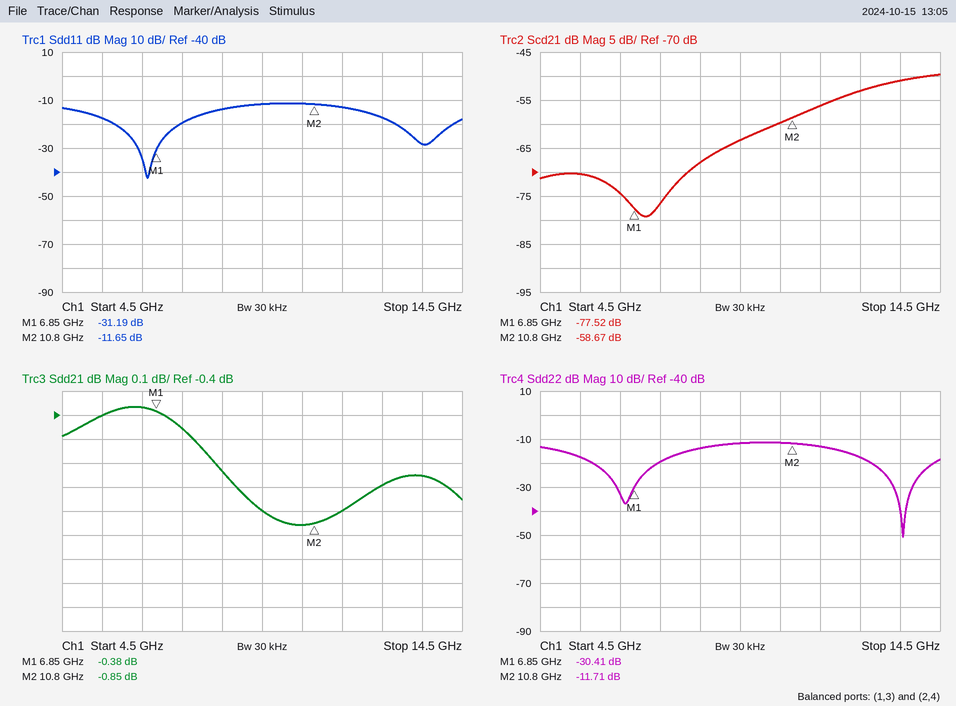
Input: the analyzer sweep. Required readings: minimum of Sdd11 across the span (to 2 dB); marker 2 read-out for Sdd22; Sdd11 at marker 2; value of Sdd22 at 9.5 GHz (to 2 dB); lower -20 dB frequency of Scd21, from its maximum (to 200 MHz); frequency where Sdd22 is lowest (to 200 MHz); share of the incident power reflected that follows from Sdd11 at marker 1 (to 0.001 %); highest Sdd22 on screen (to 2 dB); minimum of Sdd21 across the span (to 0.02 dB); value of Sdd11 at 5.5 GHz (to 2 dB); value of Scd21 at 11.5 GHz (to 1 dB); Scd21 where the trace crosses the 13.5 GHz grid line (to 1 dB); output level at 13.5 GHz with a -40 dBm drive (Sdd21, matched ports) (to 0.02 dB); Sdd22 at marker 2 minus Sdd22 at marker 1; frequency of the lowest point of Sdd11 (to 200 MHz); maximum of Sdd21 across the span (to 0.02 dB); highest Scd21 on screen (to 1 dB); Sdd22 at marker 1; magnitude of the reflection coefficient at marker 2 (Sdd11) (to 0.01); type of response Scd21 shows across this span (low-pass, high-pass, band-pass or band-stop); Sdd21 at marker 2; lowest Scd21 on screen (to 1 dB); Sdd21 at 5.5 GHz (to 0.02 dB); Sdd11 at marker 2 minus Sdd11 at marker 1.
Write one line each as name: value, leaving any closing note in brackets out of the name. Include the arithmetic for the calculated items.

minimum of Sdd11 across the span: -42 dB
marker 2 read-out for Sdd22: -11.71 dB
Sdd11 at marker 2: -11.65 dB
value of Sdd22 at 9.5 GHz: -12 dB
lower -20 dB frequency of Scd21, from its maximum: 8.2 GHz
frequency where Sdd22 is lowest: 13.6 GHz
share of the incident power reflected that follows from Sdd11 at marker 1: 10^(-31.19/10) ≈ 0.076 %
highest Sdd22 on screen: -12 dB
minimum of Sdd21 across the span: -0.86 dB
value of Sdd11 at 5.5 GHz: -18 dB
value of Scd21 at 11.5 GHz: -56 dB
Scd21 where the trace crosses the 13.5 GHz grid line: -51 dB
output level at 13.5 GHz with a -40 dBm drive (Sdd21, matched ports): -40 dBm + (-0.66 dB) = -40.66 dBm
Sdd22 at marker 2 minus Sdd22 at marker 1: -11.71 − (-30.41) = 18.70 dB
frequency of the lowest point of Sdd11: 6.6 GHz
maximum of Sdd21 across the span: -0.36 dB
highest Scd21 on screen: -50 dB
Sdd22 at marker 1: -30.41 dB
magnitude of the reflection coefficient at marker 2 (Sdd11): 10^(-11.65/20) ≈ 0.26
type of response Scd21 shows across this span: high-pass
Sdd21 at marker 2: -0.85 dB
lowest Scd21 on screen: -79 dB
Sdd21 at 5.5 GHz: -0.40 dB
Sdd11 at marker 2 minus Sdd11 at marker 1: -11.65 − (-31.19) = 19.54 dB
